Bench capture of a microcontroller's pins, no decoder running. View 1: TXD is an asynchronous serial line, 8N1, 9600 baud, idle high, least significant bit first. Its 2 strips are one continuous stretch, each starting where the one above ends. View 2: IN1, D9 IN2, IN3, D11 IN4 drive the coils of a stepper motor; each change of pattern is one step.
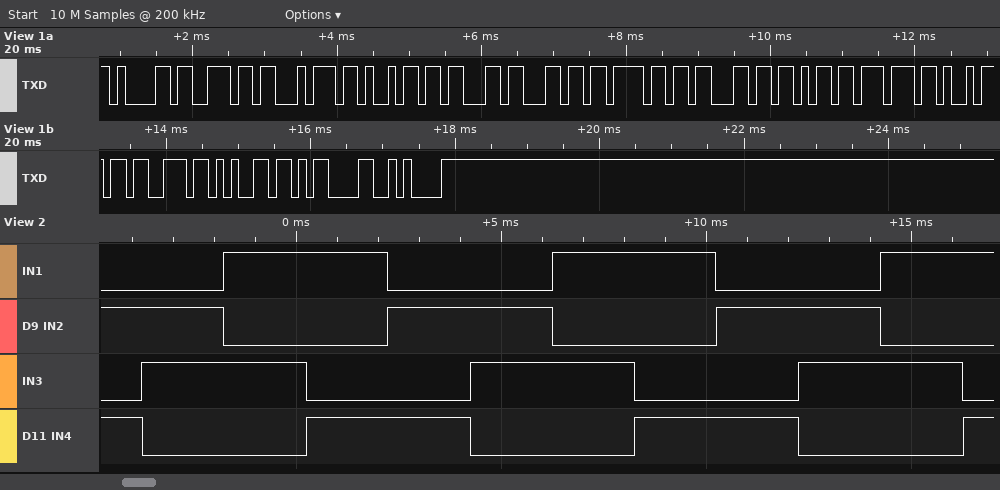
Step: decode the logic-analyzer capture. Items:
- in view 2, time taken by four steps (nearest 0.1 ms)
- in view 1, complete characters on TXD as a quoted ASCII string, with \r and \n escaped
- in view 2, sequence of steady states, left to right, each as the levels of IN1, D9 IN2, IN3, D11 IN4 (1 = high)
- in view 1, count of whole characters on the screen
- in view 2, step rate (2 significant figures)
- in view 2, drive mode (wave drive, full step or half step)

8.0 ms
"anticlockwise\r\n"
0101 0110 1010 1001 0101 0110 1010 1001 0101 0110 1010 1001
15
500 steps/s
full step
